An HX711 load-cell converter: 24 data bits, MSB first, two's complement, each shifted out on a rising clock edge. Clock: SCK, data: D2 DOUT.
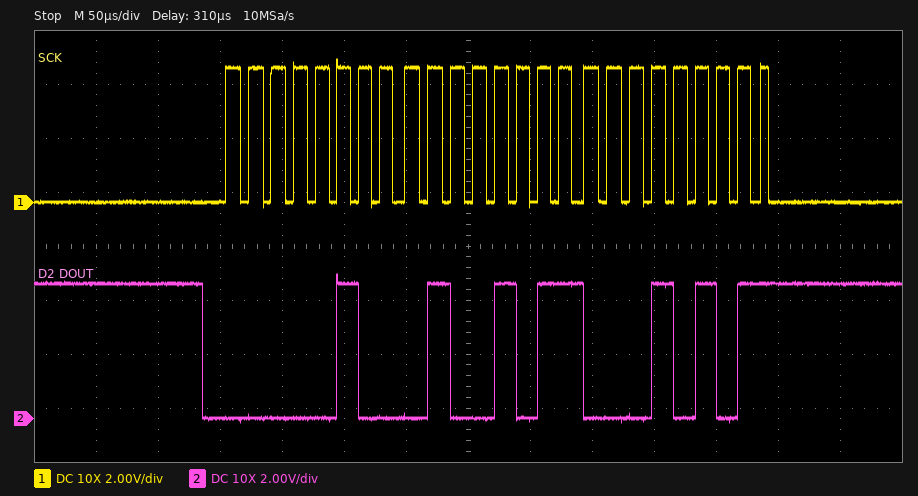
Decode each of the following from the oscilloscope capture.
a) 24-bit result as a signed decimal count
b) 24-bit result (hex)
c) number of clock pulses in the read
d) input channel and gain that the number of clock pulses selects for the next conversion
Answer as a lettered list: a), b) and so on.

a) 281365
b) 0x044B15
c) 25
d) channel A, gain 128
